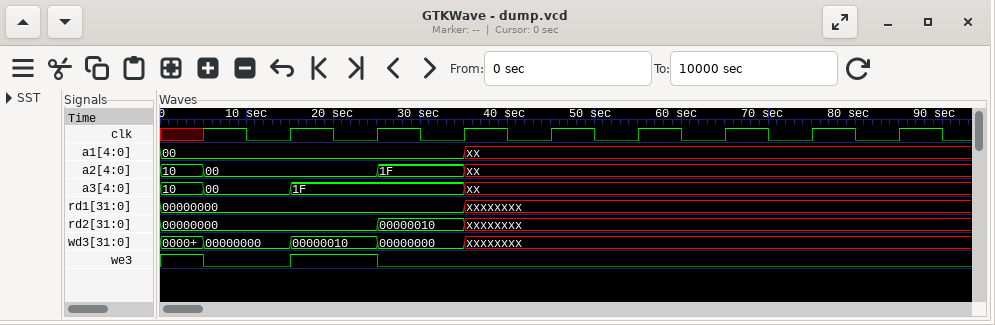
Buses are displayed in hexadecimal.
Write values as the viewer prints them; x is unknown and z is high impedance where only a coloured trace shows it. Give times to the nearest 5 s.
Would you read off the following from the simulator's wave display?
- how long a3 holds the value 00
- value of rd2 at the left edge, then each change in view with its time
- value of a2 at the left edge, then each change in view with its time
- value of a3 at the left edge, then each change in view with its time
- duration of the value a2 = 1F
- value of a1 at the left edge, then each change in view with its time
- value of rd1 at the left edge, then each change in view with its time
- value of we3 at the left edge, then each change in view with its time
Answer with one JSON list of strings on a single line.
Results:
["10 s", "00000000, 00000010 at 25 s, xxxxxxxx at 35 s", "10, 00 at 5 s, 1F at 25 s, xx at 35 s", "10, 00 at 5 s, 1F at 15 s, xx at 35 s", "10 s", "00, xx at 35 s", "00000000, xxxxxxxx at 35 s", "1, 0 at 5 s, 1 at 15 s, 0 at 25 s"]
